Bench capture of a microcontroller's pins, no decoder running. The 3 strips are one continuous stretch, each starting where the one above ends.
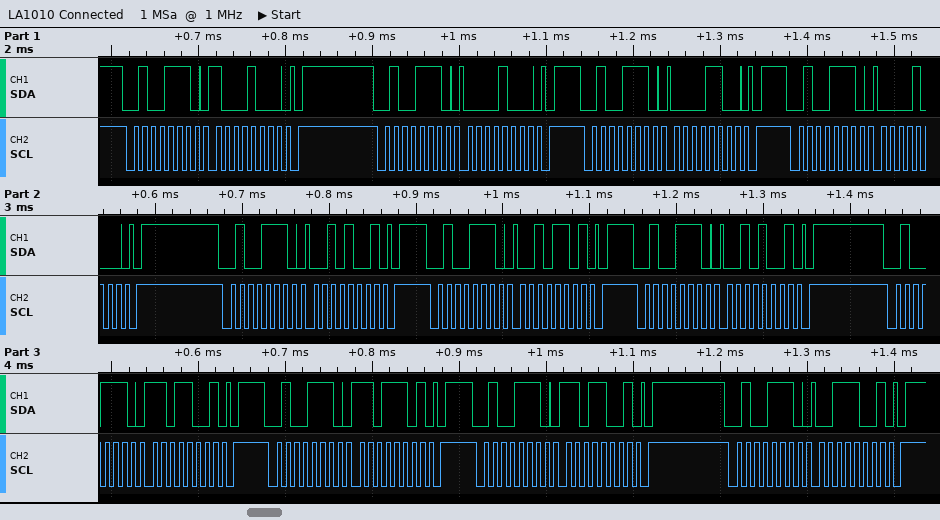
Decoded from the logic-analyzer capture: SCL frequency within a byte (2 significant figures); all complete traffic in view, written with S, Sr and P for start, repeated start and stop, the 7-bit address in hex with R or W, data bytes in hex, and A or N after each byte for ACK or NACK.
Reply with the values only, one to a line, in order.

100 kHz
S 27W A 88 A P S 27W A 08 A P S 27W A 0C A P S 27W A 08 A P S 27W A 29 A P S 27W A 2D A P S 27W A 29 A P S 27W A D9 A P S 27W A DD A P S 27W A D9 A P S 27W A 39 A P
